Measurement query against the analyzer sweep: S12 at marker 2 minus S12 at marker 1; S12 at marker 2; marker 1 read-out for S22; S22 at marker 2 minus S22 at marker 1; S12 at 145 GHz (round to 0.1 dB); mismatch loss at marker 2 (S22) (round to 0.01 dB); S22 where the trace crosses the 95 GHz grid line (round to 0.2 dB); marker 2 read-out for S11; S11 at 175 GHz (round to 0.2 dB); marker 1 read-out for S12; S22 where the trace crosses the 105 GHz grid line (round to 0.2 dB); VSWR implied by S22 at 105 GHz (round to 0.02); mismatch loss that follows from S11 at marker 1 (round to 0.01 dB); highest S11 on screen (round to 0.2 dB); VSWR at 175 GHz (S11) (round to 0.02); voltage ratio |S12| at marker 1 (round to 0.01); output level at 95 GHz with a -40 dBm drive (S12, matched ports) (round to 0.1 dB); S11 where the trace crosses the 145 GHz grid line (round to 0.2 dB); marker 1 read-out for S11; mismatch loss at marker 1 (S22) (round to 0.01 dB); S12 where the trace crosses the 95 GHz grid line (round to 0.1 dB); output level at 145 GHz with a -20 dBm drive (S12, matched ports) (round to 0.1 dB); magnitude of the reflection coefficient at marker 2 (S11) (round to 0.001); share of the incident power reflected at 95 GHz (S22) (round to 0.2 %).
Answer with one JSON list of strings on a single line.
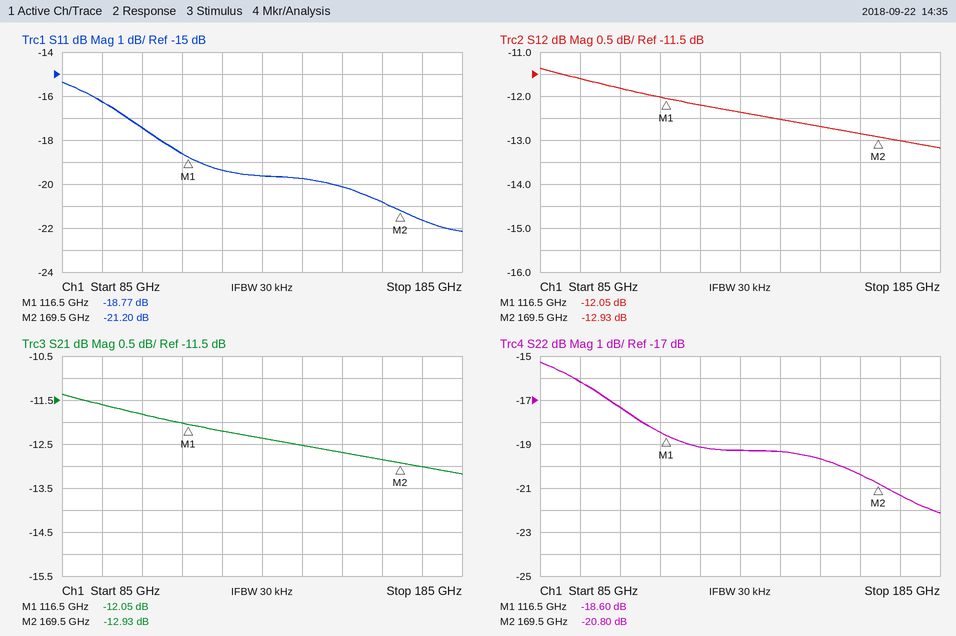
["-0.88 dB", "-12.93 dB", "-18.60 dB", "-2.20 dB", "-12.5 dB", "0.04 dB", "-16.2 dB", "-21.20 dB", "-21.6 dB", "-12.05 dB", "-17.4 dB", "1.32", "0.06 dB", "-15.4 dB", "1.18", "0.25", "-51.6 dBm", "-19.8 dB", "-18.77 dB", "0.06 dB", "-11.6 dB", "-32.5 dBm", "0.087", "2.4 %"]
